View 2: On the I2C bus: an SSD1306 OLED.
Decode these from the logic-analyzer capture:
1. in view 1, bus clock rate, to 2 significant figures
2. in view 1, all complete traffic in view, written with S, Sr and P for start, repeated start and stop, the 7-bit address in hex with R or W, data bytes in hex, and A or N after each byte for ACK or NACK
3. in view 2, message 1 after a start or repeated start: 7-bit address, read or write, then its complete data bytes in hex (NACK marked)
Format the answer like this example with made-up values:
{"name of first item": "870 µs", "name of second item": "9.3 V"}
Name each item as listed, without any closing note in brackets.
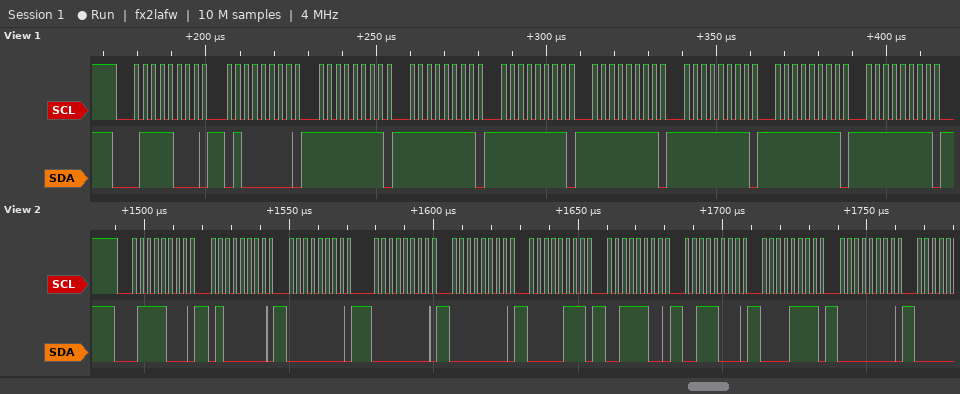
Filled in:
{"in view 1, bus clock rate, to 2 significant figures": "400 kHz", "in view 1, all complete traffic in view, written with S, Sr and P for start, repeated start and stop, the 7-bit address in hex with R or W, data bytes in hex, and A or N after each byte for ACK or NACK": "S 3CW A 40 A FF A FF A FF A FF A FF A FF A FF A", "in view 2, message 1 after a start or repeated start: 7-bit address, read or write, then its complete data bytes in hex": "0x3C write: 40 00 00 00 07 3C 38 0F 00"}
